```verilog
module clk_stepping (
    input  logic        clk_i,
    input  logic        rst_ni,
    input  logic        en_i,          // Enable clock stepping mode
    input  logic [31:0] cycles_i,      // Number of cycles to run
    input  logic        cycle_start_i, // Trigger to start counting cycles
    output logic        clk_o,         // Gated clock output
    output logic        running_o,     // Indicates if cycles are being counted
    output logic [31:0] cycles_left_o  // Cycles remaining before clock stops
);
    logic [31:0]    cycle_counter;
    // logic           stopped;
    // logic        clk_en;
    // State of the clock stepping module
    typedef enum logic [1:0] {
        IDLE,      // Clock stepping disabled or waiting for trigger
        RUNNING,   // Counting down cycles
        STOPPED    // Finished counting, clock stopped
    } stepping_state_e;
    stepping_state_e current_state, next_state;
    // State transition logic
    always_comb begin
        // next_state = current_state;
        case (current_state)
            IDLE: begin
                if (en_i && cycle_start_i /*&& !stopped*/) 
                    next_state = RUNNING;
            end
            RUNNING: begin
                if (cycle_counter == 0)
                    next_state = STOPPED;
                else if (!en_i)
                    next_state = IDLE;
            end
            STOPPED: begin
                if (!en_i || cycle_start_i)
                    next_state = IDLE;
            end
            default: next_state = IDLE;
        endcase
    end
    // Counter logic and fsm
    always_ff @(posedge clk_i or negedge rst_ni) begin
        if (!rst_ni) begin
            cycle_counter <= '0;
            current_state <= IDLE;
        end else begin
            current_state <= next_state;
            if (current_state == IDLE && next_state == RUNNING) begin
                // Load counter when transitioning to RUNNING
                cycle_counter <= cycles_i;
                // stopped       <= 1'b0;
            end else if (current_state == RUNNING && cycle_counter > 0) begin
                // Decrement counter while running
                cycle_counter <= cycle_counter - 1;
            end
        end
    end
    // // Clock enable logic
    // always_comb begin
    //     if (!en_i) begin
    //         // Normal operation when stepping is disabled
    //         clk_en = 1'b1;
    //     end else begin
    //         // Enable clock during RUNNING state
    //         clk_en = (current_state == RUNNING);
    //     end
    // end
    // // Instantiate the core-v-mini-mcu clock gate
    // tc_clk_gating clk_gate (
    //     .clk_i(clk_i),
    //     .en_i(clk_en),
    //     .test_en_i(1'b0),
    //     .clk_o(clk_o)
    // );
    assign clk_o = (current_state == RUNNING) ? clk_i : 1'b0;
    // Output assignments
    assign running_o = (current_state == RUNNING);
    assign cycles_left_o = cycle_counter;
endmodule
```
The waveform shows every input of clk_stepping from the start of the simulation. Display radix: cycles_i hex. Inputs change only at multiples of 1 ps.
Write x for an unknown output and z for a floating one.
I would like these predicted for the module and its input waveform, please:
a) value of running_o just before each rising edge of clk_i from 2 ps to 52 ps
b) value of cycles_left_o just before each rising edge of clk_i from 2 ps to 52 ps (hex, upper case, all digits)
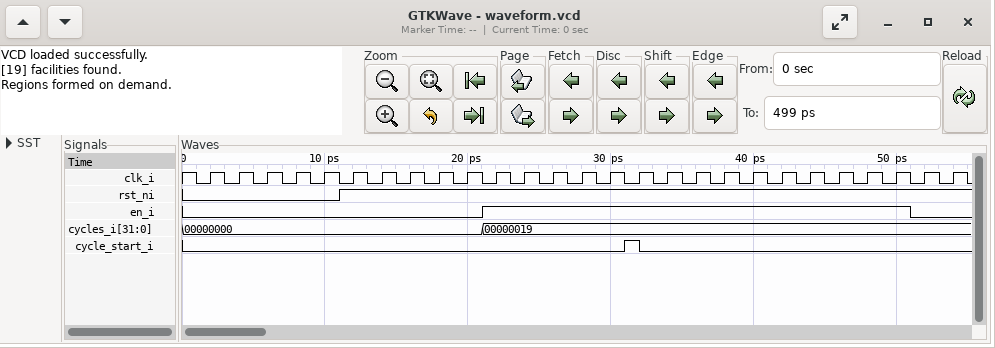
0 0 0 0 0 0 0 0 0 0 0 0 0 0 0 0 1 1 1 1 1 1 1 1 1 1
00000000, 00000000, 00000000, 00000000, 00000000, 00000000, 00000000, 00000000, 00000000, 00000000, 00000000, 00000000, 00000000, 00000000, 00000000, 00000000, 00000019, 00000018, 00000017, 00000016, 00000015, 00000014, 00000013, 00000012, 00000011, 00000010
